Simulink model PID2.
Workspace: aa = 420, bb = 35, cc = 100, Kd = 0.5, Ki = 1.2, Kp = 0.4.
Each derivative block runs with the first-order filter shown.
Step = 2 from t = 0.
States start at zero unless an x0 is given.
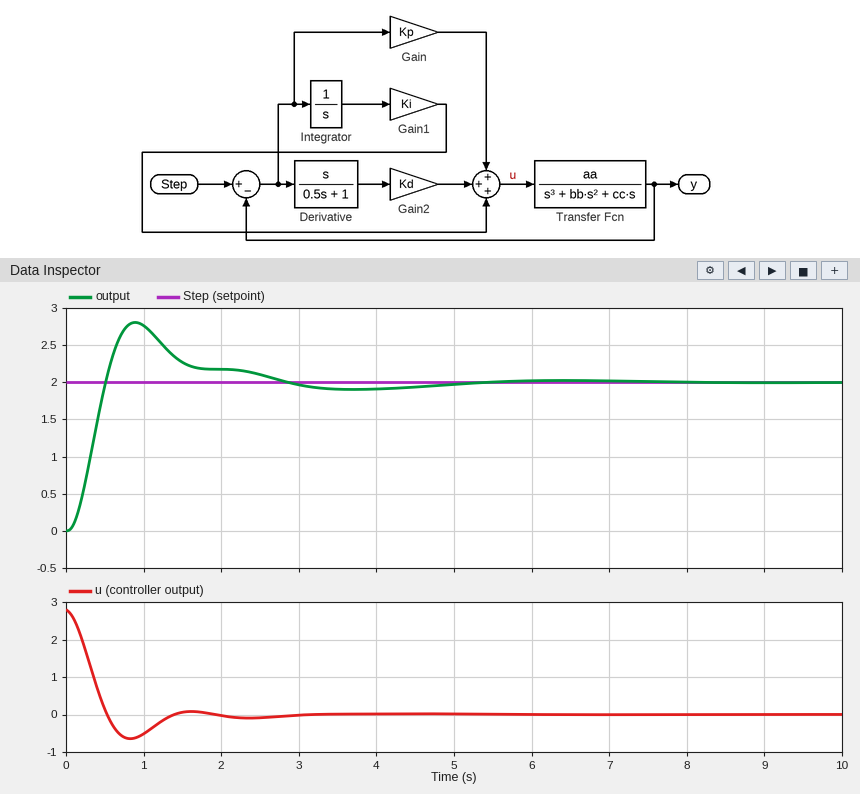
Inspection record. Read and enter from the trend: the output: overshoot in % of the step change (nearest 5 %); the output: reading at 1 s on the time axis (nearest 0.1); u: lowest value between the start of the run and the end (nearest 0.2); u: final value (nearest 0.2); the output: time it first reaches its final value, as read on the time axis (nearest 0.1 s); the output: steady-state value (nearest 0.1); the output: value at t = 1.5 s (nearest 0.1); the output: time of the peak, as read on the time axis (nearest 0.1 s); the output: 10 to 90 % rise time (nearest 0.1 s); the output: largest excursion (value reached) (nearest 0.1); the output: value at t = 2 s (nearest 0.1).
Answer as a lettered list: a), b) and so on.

a) 40 %
b) 2.8
c) -0.6
d) 0.0
e) 0.5 s
f) 2.0
g) 2.3
h) 0.9 s
i) 0.3 s
j) 2.8
k) 2.2
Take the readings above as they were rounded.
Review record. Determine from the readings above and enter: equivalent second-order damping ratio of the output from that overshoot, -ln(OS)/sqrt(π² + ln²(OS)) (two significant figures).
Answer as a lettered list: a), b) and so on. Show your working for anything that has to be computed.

a) ln(0.4) = -0.916; 0.916 / sqrt(9.870 + 0.840) = 0.28
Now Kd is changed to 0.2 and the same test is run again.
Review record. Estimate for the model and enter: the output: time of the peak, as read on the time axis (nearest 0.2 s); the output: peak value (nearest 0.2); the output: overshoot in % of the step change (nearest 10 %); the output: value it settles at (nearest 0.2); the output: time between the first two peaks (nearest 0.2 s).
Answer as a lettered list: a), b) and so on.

a) 1.2 s
b) 3.4
c) 70 %
d) 2.0
e) 3.0 s
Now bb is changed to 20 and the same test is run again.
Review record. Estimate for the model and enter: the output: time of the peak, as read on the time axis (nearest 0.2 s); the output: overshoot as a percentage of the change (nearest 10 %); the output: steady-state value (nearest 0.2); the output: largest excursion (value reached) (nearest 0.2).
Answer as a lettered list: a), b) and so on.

a) 0.6 s
b) 30 %
c) 2.0
d) 2.6
